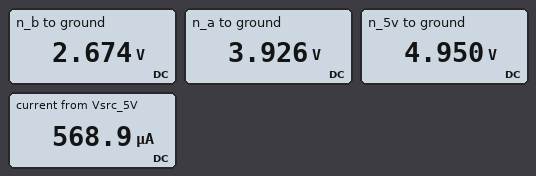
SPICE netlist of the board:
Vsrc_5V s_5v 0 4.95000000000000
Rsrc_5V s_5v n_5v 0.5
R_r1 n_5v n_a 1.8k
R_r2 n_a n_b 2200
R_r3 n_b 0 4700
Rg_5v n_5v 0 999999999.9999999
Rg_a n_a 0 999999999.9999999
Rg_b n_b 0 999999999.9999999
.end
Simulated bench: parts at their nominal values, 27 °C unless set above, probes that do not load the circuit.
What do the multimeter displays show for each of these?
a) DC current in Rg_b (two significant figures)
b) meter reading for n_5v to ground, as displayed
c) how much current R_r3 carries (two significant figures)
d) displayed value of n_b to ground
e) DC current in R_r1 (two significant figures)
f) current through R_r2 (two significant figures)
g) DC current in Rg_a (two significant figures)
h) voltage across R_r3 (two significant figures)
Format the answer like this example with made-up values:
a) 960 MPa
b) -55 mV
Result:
a) 2.7 nA
b) 4.950 V
c) 570 µA
d) 2.674 V
e) 570 µA
f) 570 µA
g) 3.9 nA
h) 2.7 V
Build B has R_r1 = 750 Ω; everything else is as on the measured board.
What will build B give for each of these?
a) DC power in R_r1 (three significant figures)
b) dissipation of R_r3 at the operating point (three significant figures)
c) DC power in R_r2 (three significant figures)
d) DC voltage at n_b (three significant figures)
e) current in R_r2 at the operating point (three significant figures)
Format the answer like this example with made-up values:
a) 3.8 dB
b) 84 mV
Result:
a) 314 µW
b) 1.97 mW
c) 921 µW
d) 3.04 V
e) 647 µA
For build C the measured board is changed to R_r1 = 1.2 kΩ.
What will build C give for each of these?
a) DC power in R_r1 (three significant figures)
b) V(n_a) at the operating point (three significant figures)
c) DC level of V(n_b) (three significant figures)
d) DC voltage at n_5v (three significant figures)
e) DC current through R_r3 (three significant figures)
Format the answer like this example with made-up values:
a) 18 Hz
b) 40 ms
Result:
a) 448 µW
b) 4.22 V
c) 2.87 V
d) 4.95 V
e) 611 µA
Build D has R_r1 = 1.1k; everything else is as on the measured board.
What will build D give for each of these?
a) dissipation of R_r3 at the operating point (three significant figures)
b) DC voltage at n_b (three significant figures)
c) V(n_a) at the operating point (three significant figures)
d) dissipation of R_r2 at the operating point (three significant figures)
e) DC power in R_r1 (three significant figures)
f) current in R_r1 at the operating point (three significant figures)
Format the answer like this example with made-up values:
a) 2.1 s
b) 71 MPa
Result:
a) 1.80 mW
b) 2.91 V
c) 4.27 V
d) 842 µW
e) 421 µW
f) 619 µA
